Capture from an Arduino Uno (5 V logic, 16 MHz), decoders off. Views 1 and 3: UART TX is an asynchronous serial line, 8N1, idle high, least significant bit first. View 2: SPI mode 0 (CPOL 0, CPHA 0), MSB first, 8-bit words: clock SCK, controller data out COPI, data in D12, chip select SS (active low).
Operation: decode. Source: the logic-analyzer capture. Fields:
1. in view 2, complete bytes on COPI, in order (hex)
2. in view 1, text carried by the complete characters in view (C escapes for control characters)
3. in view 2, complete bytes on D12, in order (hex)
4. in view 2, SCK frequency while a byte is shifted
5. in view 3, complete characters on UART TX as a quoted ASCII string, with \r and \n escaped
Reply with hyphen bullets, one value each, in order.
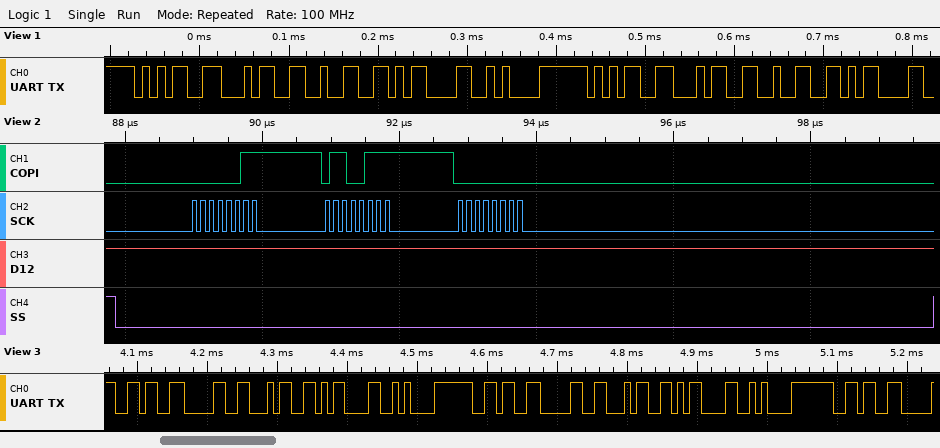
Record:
- 03 67 00
- "542\r\n542\r"
- FF FF FF
- 8 MHz
- "604\r\n604\r\n6"
